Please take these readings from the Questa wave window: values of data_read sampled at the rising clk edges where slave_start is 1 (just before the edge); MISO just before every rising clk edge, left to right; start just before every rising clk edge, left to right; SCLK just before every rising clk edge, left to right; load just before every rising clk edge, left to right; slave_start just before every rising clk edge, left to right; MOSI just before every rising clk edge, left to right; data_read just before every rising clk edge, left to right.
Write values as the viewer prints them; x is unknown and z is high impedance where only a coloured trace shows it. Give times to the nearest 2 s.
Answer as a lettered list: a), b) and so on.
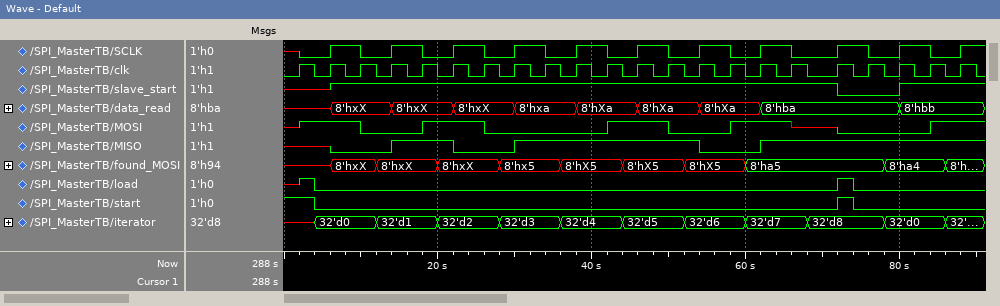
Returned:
a) 8'hxX, 8'hxX, 8'hxX, 8'hxX, 8'hxX, 8'hxX, 8'hxa, 8'hxa, 8'hXa, 8'hXa, 8'hXa, 8'hXa, 8'hXa, 8'hXa, 8'hba, 8'hba, 8'hbb, 8'hbb
b) x x 0 0 1 1 0 0 1 1 1 1 1 1 0 0 1 1 1 1 1 1
c) 1 0 0 0 0 0 0 0 0 0 0 0 0 0 0 0 0 0 0 0 0 0
d) x 0 1 0 1 0 1 0 1 0 1 0 1 0 1 0 1 0 1 0 1 0
e) x 0 0 0 0 0 0 0 0 0 0 0 0 0 0 0 0 0 0 0 0 0
f) x x 1 1 1 1 1 1 1 1 1 1 1 1 1 1 1 1 0 0 1 1
g) x 1 1 0 0 1 1 0 0 0 0 1 1 0 0 1 1 x 0 0 0 1
h) x, x, 8'hxX, 8'hxX, 8'hxX, 8'hxX, 8'hxX, 8'hxX, 8'hxa, 8'hxa, 8'hXa, 8'hXa, 8'hXa, 8'hXa, 8'hXa, 8'hXa, 8'hba, 8'hba, 8'hba, 8'hba, 8'hbb, 8'hbb
